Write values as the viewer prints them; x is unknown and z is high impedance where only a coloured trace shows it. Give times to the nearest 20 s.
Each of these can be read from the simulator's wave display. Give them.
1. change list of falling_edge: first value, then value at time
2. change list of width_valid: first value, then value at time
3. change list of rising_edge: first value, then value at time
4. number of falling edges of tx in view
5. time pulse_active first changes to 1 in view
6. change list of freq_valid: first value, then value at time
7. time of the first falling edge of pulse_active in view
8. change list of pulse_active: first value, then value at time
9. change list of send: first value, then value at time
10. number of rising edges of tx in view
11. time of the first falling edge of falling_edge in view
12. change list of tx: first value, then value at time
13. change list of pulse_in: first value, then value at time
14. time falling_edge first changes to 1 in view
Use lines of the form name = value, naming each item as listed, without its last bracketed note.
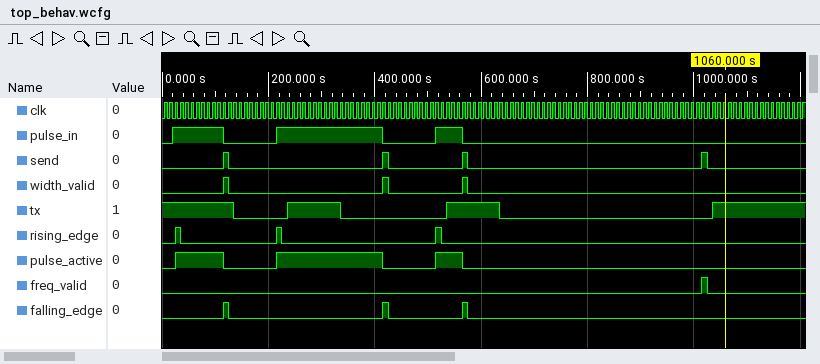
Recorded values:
change list of falling_edge: first value, then value at time = 0, 1 at 120 s, 0 at 120 s, 1 at 420 s, 0 at 420 s, 1 at 560 s, 0 at 580 s
change list of width_valid: first value, then value at time = 0, 1 at 120 s, 0 at 120 s, 1 at 420 s, 0 at 420 s, 1 at 560 s, 0 at 580 s
change list of rising_edge: first value, then value at time = 0, 1 at 20 s, 0 at 40 s, 1 at 220 s, 0 at 220 s, 1 at 520 s, 0 at 520 s
number of falling edges of tx in view = 3
time pulse_active first changes to 1 in view = 20 s
change list of freq_valid: first value, then value at time = 0, 1 at 1020 s, 0 at 1020 s
time of the first falling edge of pulse_active in view = 120 s
change list of pulse_active: first value, then value at time = 0, 1 at 20 s, 0 at 120 s, 1 at 220 s, 0 at 420 s, 1 at 520 s, 0 at 560 s
change list of send: first value, then value at time = 0, 1 at 120 s, 0 at 120 s, 1 at 420 s, 0 at 420 s, 1 at 560 s, 0 at 580 s, 1 at 1020 s, 0 at 1020 s
number of rising edges of tx in view = 3
time of the first falling edge of falling_edge in view = 120 s
change list of tx: first value, then value at time = 1, 0 at 140 s, 1 at 240 s, 0 at 340 s, 1 at 540 s, 0 at 640 s, 1 at 1040 s
change list of pulse_in: first value, then value at time = 0, 1 at 20 s, 0 at 120 s, 1 at 220 s, 0 at 420 s, 1 at 520 s, 0 at 560 s
time falling_edge first changes to 1 in view = 120 s
